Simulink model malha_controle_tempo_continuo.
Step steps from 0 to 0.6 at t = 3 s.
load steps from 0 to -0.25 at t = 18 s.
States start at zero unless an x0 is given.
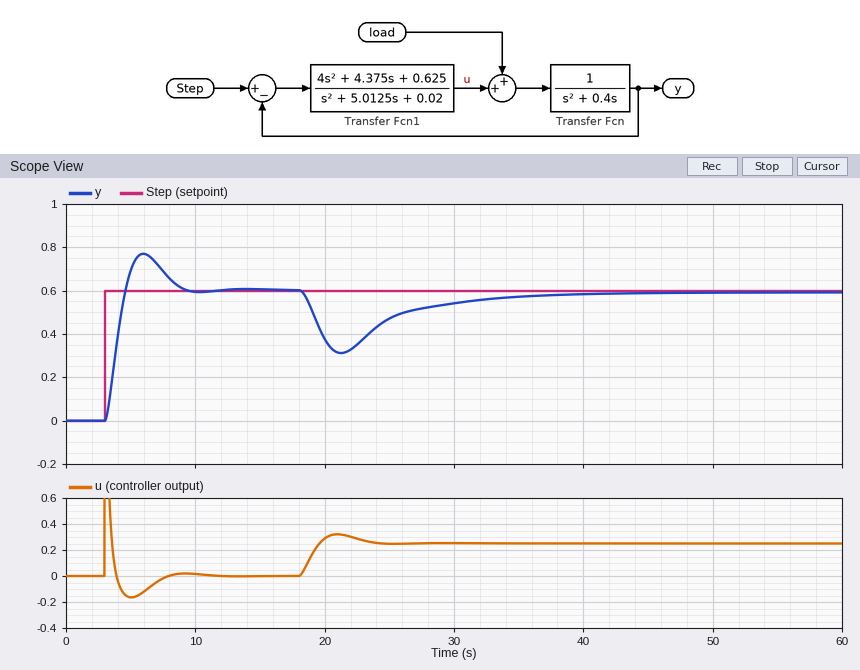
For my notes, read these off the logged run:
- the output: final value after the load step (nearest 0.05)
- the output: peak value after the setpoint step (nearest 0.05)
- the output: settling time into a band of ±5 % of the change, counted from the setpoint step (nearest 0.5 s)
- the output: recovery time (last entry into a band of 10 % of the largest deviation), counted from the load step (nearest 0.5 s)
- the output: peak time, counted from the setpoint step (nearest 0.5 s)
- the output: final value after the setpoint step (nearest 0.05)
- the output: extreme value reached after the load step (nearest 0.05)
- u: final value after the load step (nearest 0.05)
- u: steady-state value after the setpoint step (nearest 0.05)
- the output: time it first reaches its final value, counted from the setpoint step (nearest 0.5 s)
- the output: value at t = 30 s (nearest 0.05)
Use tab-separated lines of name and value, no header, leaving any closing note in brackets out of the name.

the output: final value after the load step	0.60
the output: peak value after the setpoint step	0.75
the output: settling time into a band of ±5 % of the change, counted from the setpoint step	5.5 s
the output: recovery time (last entry into a band of 10 % of the largest deviation), counted from the load step	15.0 s
the output: peak time, counted from the setpoint step	3.0 s
the output: final value after the setpoint step	0.60
the output: extreme value reached after the load step	0.30
u: final value after the load step	0.25
u: steady-state value after the setpoint step	0.00
the output: time it first reaches its final value, counted from the setpoint step	1.5 s
the output: value at t = 30 s	0.55
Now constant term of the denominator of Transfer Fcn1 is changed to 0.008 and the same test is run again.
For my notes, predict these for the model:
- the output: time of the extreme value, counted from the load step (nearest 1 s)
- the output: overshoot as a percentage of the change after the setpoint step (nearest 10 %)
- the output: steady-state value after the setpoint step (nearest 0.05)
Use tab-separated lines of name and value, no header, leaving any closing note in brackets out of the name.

the output: time of the extreme value, counted from the load step	3 s
the output: overshoot as a percentage of the change after the setpoint step	30 %
the output: steady-state value after the setpoint step	0.60
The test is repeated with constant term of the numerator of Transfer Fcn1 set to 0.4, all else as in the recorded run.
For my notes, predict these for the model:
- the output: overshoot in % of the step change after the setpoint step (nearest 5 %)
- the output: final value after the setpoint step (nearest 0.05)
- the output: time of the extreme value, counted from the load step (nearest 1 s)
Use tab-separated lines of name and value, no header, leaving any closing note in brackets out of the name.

the output: overshoot in % of the step change after the setpoint step	25 %
the output: final value after the setpoint step	0.60
the output: time of the extreme value, counted from the load step	3 s
